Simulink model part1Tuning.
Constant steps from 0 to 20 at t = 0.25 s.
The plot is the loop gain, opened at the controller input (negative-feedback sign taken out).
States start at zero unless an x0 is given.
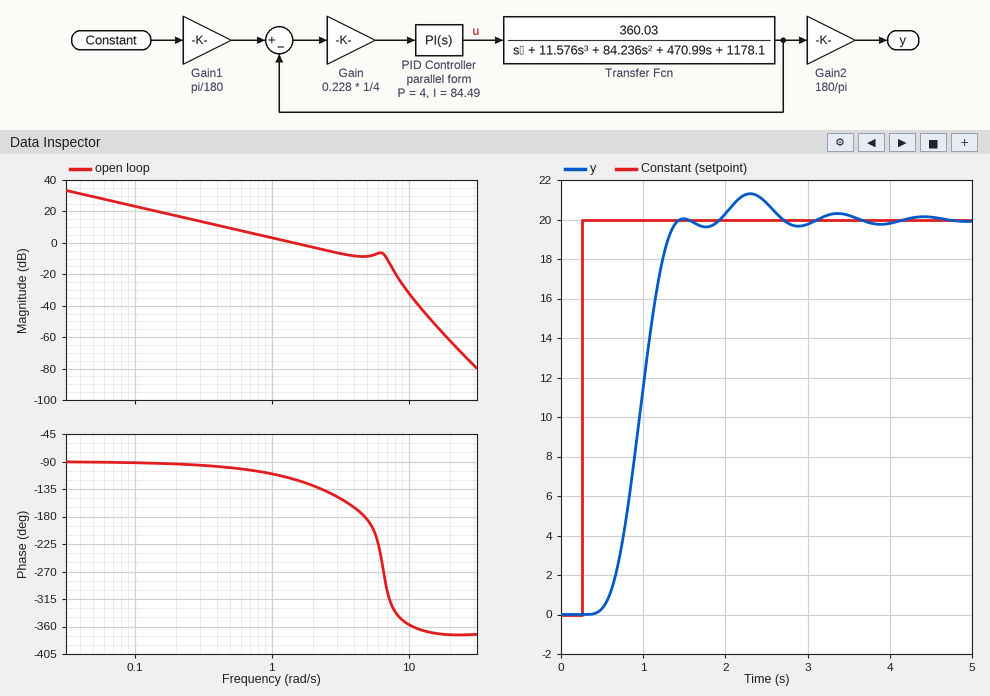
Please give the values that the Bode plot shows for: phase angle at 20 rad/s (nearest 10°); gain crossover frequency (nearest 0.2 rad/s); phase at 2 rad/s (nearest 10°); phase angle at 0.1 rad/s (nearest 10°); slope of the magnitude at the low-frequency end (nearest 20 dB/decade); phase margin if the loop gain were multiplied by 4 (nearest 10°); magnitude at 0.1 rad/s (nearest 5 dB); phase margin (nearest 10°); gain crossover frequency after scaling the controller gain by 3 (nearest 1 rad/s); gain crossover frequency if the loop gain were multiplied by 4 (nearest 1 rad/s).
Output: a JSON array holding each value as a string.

["-370°", "1.4 rad/s", "-130°", "-90°", "-20 dB/decade", "-130°", "25 dB", "60°", "7 rad/s", "7 rad/s"]
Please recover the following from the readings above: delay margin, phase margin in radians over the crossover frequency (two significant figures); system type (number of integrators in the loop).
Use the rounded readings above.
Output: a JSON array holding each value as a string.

["0.75 s", "1"]
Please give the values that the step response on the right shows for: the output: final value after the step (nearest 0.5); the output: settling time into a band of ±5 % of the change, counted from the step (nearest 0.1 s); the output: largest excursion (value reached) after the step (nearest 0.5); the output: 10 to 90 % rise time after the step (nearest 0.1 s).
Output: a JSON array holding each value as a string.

["20.0", "2.2 s", "21.5", "0.6 s"]
